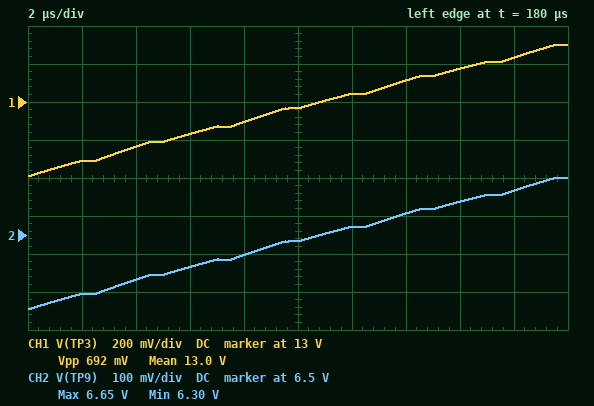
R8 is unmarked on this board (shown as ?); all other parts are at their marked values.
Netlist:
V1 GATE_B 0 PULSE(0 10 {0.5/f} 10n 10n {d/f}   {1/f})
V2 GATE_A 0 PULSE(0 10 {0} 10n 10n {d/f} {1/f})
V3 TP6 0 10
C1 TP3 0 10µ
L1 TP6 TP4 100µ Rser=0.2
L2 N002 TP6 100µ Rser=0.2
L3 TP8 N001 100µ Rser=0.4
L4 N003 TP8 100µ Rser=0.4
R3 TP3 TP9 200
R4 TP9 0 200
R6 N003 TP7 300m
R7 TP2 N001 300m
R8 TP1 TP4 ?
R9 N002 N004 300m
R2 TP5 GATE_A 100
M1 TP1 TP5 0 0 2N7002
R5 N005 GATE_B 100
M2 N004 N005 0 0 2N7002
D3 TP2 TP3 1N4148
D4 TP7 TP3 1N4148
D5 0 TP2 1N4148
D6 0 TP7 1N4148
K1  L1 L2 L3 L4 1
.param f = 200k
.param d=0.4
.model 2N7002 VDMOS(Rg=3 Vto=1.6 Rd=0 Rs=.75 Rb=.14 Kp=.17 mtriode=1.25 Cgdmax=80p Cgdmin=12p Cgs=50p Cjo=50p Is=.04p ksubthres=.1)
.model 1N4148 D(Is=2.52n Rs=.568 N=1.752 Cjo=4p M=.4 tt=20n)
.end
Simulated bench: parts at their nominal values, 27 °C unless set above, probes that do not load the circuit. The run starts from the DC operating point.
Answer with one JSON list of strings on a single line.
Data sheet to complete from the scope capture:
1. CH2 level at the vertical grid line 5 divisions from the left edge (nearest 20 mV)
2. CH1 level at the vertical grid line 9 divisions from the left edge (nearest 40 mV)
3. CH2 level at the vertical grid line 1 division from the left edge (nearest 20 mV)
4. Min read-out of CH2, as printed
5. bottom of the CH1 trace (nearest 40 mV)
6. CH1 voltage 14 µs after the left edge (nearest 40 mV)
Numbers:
["6.48 V", "13.24 V", "6.34 V", "6.30 V", "12.60 V", "13.12 V"]
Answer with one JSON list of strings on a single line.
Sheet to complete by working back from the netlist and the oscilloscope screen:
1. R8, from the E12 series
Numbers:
["1 Ω"]
